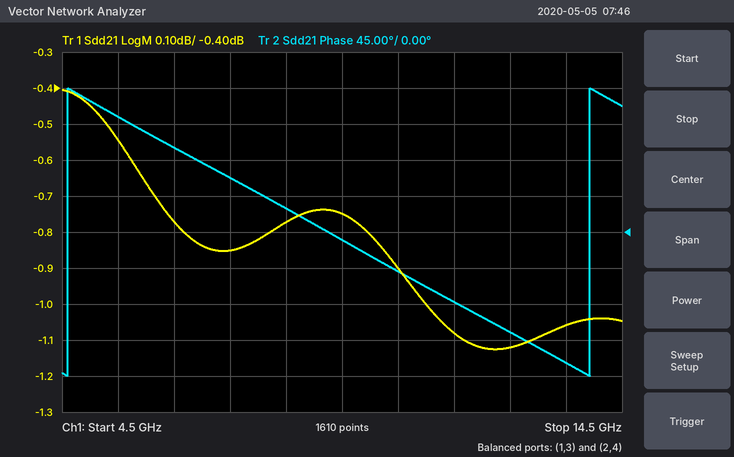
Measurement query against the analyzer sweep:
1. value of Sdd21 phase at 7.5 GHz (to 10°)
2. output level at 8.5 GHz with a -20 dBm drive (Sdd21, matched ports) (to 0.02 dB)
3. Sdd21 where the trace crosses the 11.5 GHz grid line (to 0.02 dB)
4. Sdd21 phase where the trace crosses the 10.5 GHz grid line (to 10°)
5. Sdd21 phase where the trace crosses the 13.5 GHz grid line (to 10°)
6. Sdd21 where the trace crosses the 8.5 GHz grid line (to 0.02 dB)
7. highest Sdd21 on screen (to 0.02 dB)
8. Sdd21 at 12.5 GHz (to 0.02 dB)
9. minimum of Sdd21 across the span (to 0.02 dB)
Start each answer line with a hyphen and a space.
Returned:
- 70°
- -20.78 dBm
- -1.08 dB
- -50°
- -160°
- -0.78 dB
- -0.40 dB
- -1.12 dB
- -1.12 dB
